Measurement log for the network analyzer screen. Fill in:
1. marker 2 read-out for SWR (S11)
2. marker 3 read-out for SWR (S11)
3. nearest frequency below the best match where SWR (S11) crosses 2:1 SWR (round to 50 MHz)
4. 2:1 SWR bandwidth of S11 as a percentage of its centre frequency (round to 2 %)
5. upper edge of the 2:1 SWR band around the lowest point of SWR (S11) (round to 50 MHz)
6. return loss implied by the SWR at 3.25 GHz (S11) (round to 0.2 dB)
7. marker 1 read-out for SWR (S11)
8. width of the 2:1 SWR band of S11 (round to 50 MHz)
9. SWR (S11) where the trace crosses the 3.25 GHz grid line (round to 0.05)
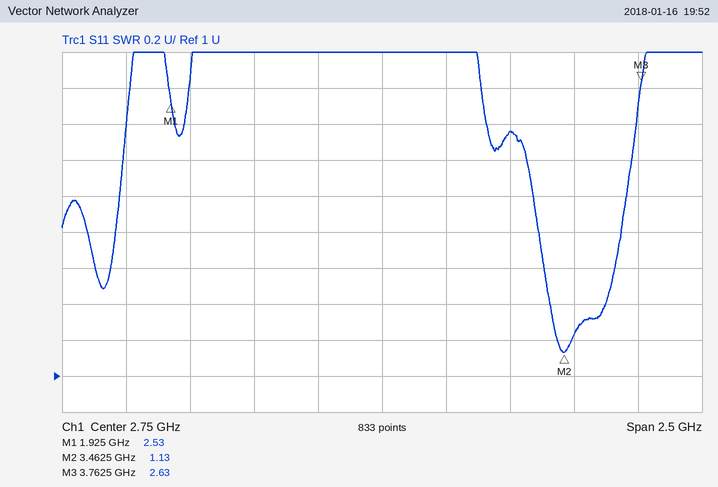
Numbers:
1.13
2.63
3.35 GHz
10 %
3.70 GHz
7.8 dB
2.53
350 MHz
2.35
